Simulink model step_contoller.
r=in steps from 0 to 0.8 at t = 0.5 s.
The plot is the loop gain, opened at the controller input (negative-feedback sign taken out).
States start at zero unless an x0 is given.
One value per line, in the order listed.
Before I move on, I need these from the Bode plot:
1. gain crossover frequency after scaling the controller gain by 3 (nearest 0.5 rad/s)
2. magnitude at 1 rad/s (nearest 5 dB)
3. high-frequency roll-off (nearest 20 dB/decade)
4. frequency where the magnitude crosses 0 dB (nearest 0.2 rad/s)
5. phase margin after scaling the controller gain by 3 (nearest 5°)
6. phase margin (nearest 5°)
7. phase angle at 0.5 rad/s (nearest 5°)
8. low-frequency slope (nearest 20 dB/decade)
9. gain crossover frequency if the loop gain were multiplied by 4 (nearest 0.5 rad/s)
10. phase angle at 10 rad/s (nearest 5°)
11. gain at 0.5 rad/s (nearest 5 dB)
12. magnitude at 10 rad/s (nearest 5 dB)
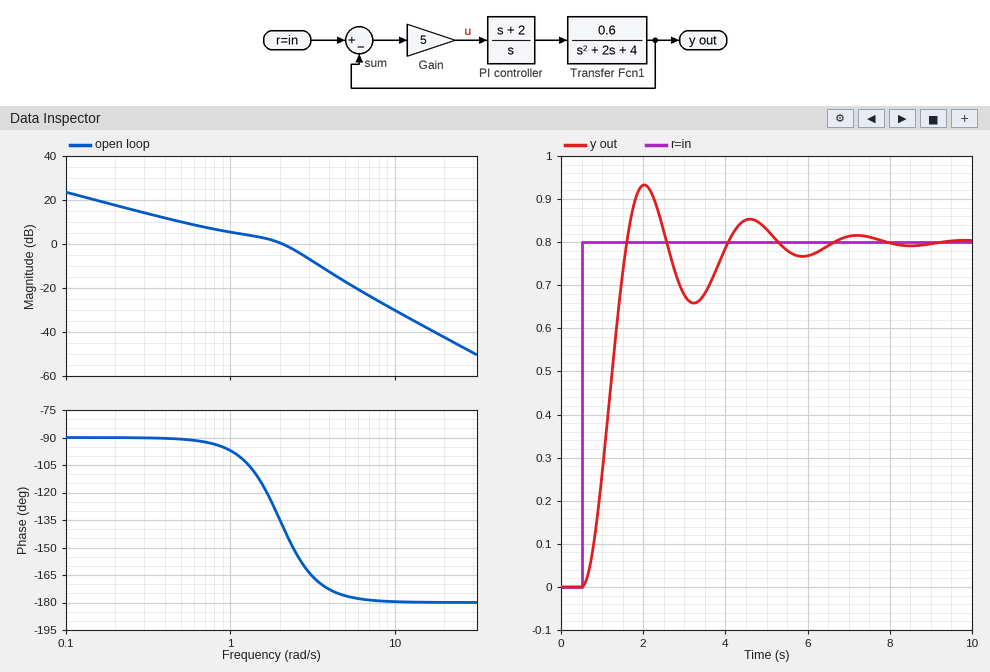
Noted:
3.5 rad/s
5 dB
-40 dB/decade
2.0 rad/s
10°
40°
-90°
-20 dB/decade
4.0 rad/s
-180°
10 dB
-30 dB
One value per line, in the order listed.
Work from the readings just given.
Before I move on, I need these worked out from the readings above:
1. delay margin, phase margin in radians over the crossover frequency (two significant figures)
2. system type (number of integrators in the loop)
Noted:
0.35 s
1
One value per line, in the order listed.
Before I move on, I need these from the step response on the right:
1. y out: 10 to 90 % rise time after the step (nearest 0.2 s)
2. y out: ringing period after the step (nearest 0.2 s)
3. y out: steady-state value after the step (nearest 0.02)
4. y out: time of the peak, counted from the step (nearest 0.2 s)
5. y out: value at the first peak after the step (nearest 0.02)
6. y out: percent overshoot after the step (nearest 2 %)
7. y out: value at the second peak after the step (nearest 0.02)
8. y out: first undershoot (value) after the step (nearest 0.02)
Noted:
0.8 s
2.6 s
0.80
1.6 s
0.94
16 %
0.86
0.66
